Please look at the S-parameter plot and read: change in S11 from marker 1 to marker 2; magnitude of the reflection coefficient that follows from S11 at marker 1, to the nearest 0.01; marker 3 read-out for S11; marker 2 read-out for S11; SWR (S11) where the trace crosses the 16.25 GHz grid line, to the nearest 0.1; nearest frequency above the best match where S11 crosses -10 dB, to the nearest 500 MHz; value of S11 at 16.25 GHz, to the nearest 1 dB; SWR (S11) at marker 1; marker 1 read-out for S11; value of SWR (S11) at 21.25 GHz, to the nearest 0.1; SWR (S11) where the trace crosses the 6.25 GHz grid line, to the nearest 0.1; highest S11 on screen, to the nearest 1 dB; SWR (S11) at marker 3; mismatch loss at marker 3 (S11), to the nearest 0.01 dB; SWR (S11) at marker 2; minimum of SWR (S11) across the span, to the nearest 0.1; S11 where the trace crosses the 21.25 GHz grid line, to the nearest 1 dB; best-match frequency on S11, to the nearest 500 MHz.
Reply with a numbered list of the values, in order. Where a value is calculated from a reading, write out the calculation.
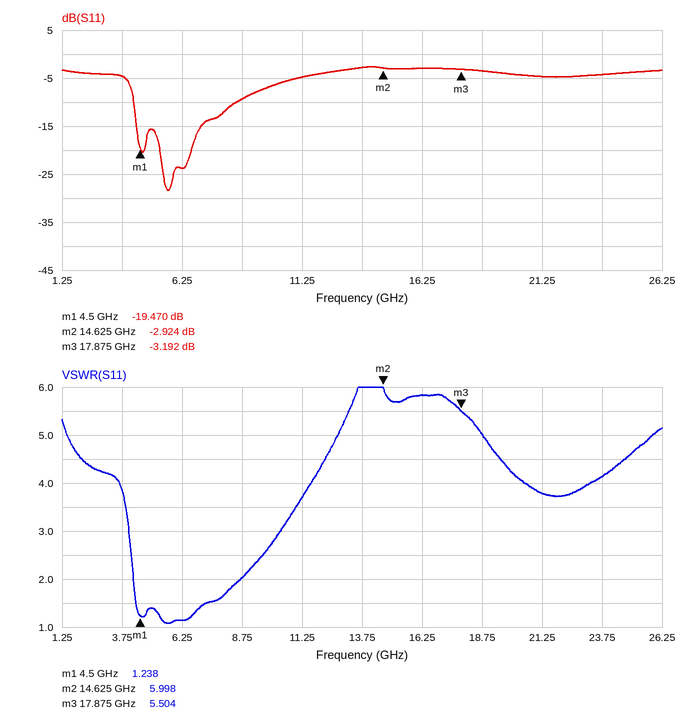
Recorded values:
1. -2.924 − (-19.47) = 16.546 dB
2. 10^(-19.47/20) ≈ 0.11
3. -3.192 dB
4. -2.924 dB
5. 5.8
6. 8.5 GHz
7. -3 dB
8. 1.238
9. -19.470 dB
10. 3.8
11. 1.1
12. -3 dB
13. 5.504
14. −10 log10(1 − 10^(-3.192/10)) ≈ 2.84 dB
15. 5.998
16. 1.1
17. -5 dB
18. 5.5 GHz
